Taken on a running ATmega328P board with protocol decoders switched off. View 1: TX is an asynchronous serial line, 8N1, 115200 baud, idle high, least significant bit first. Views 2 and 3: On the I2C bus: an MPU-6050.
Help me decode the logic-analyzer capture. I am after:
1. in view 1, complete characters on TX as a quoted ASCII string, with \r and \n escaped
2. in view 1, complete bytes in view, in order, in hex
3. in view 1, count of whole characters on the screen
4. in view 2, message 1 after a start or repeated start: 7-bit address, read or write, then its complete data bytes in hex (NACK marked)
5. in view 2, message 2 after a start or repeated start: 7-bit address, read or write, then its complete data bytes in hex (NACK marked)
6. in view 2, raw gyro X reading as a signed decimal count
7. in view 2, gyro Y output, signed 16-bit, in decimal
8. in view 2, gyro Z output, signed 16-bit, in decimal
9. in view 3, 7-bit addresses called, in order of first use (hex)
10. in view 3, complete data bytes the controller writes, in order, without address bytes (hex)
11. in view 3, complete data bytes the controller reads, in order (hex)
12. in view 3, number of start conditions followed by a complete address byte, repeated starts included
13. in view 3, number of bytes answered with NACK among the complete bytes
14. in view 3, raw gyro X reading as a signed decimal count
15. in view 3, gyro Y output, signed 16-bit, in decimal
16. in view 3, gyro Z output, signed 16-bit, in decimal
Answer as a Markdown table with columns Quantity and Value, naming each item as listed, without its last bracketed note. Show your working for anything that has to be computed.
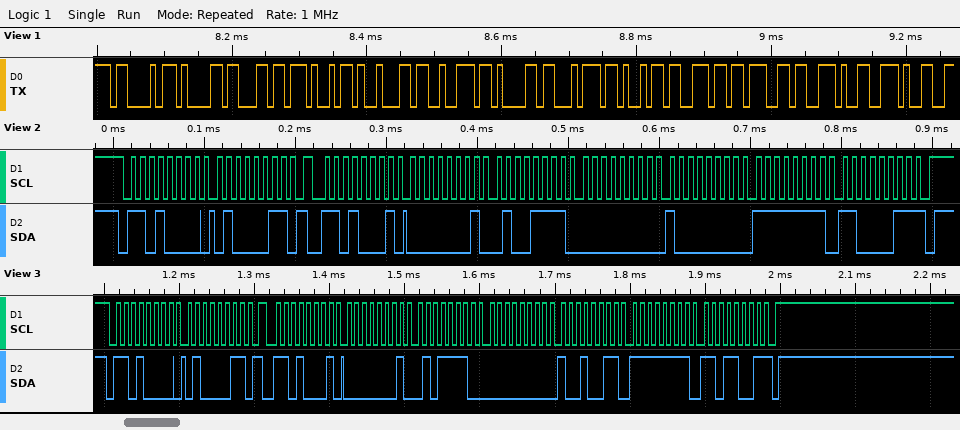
| Quantity | Value |
|---|---|
| in view 1, complete characters on TX as a quoted ASCII string, with \r and \n escaped | "Calibrating.." |
| in view 1, complete bytes in view, in order, in hex | 43 61 6C 69 62 72 61 74 69 6E 67 2E 2E |
| in view 1, count of whole characters on the screen | 13 |
| in view 2, message 1 after a start or repeated start: 7-bit address, read or write, then its complete data bytes in hex | 0x68 write: 43 |
| in view 2, message 2 after a start or repeated start: 7-bit address, read or write, then its complete data bytes in hex | 0x68 read: 01 4F 00 80 FF C3 NACK |
| in view 2, raw gyro X reading as a signed decimal count | 0x014F = 335 |
| in view 2, gyro Y output, signed 16-bit, in decimal | 0x0080 = 128 |
| in view 2, gyro Z output, signed 16-bit, in decimal | 0xFFC3 = -61 |
| in view 3, 7-bit addresses called, in order of first use | 0x68 |
| in view 3, complete data bytes the controller writes, in order, without address bytes | 43 |
| in view 3, complete data bytes the controller reads, in order | 01 5E 00 93 FF D9 |
| in view 3, number of start conditions followed by a complete address byte, repeated starts included | 2 |
| in view 3, number of bytes answered with NACK among the complete bytes | 1 |
| in view 3, raw gyro X reading as a signed decimal count | 0x015E = 350 |
| in view 3, gyro Y output, signed 16-bit, in decimal | 0x0093 = 147 |
| in view 3, gyro Z output, signed 16-bit, in decimal | 0xFFD9 = -39 |
